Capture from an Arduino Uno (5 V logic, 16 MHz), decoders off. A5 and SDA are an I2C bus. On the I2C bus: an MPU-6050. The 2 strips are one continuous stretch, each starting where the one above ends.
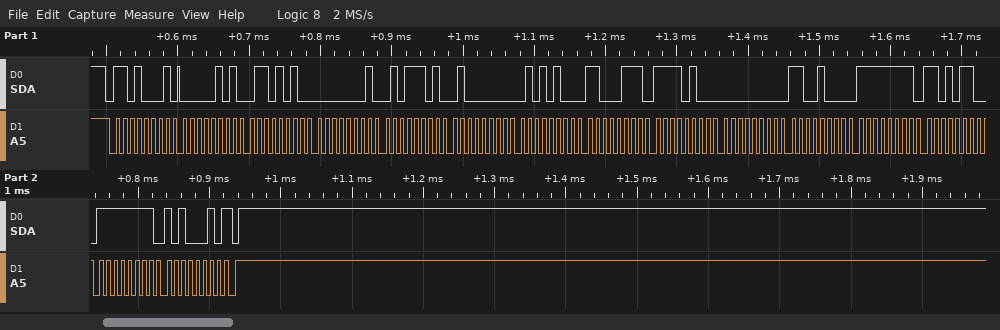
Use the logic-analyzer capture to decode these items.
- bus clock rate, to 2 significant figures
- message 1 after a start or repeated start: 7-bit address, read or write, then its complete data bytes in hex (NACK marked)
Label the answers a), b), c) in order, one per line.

a) 100 kHz
b) 0x68 read: 05 6A 01 5D 40 54 C7 F4 00 C8 FF D6 FF A2 NACK
